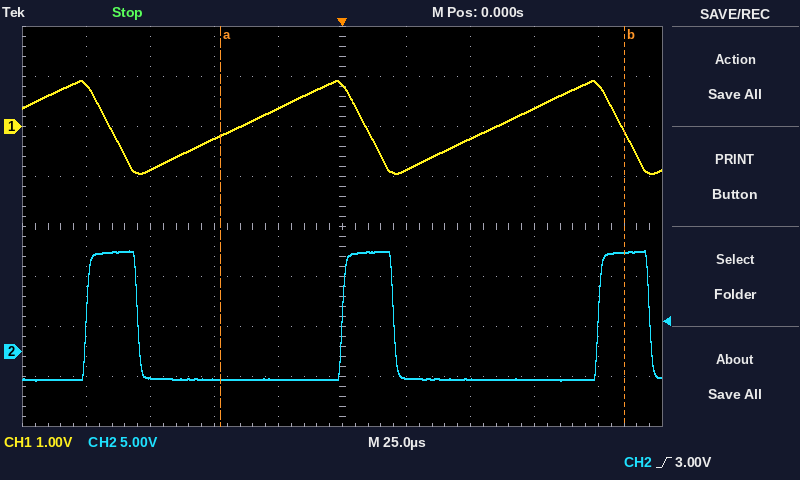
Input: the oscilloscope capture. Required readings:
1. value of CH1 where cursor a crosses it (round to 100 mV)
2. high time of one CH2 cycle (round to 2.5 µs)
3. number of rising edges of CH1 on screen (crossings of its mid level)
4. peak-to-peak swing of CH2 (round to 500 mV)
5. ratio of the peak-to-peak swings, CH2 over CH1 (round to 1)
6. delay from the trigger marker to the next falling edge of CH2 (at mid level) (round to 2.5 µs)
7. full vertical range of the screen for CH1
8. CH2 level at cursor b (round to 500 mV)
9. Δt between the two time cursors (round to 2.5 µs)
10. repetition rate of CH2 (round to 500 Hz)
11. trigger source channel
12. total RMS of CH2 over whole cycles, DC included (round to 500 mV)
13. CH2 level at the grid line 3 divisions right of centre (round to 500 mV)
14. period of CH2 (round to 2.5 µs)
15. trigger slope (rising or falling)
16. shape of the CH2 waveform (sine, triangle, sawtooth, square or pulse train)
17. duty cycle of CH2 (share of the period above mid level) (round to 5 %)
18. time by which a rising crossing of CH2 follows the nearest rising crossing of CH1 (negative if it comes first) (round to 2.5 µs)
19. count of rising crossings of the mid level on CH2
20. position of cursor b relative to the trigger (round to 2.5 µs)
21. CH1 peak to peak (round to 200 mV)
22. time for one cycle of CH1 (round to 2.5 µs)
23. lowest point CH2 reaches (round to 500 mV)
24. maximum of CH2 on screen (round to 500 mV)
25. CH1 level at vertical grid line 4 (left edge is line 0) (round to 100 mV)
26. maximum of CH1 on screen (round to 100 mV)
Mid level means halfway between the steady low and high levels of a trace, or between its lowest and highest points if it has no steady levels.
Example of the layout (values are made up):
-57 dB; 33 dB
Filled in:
-200 mV; 20.0 µs; 2; 13.0 V; 7; 20.0 µs; 8 V; 10.0 V; 157.5 µs; 10.0 kHz; CH2; 5.0 V; -3.0 V; 100.0 µs; rising; pulse train; 20 %; +40.0 µs; 3; +110.0 µs; 1.8 V; 100.0 µs; -3.0 V; 10.0 V; 400 mV; 900 mV
